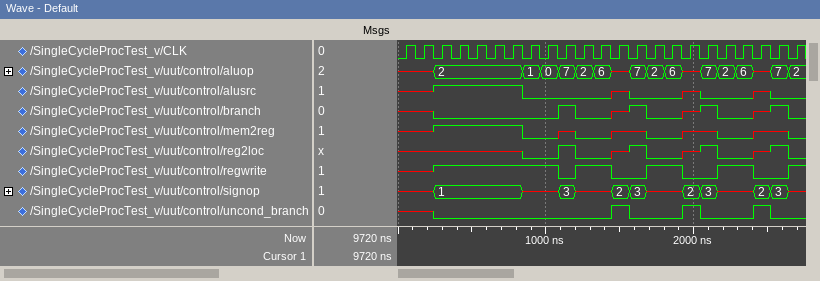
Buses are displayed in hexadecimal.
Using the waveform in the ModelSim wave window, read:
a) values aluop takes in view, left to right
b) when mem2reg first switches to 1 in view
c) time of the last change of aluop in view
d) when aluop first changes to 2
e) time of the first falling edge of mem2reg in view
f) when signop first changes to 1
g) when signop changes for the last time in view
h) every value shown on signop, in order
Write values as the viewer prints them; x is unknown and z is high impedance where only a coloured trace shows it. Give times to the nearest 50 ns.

x, 2, 1, 0, 7, 2, 6, x, 7, 2, 6, x, 7, 2, 6, x, 7, 2
250 ns
2650 ns
250 ns
850 ns
250 ns
2650 ns
x, 1, x, 3, x, 2, 3, x, 2, 3, x, 2, 3, x
